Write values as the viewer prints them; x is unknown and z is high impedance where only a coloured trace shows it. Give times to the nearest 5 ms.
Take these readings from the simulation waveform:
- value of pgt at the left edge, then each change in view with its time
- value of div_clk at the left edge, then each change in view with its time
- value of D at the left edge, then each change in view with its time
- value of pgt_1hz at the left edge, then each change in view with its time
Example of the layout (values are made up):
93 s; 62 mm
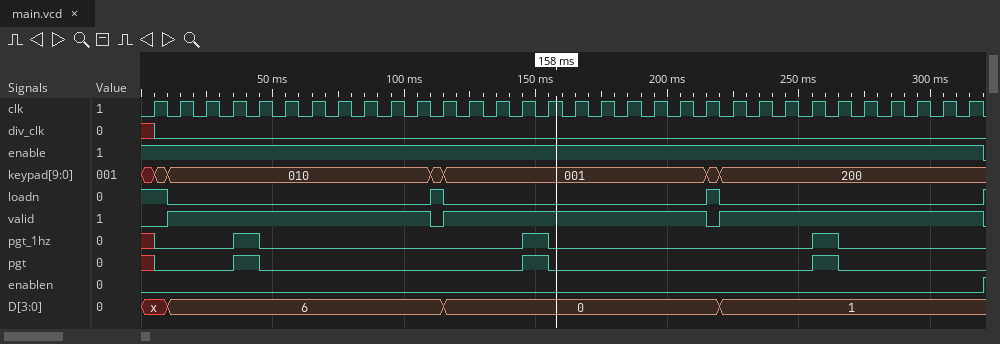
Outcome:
x, 0 at 5 ms, 1 at 35 ms, 0 at 45 ms, 1 at 145 ms, 0 at 155 ms, 1 at 255 ms, 0 at 265 ms; x, 0 at 5 ms; x, 6 at 10 ms, 0 at 115 ms, 1 at 220 ms; x, 0 at 5 ms, 1 at 35 ms, 0 at 45 ms, 1 at 145 ms, 0 at 155 ms, 1 at 255 ms, 0 at 265 ms
